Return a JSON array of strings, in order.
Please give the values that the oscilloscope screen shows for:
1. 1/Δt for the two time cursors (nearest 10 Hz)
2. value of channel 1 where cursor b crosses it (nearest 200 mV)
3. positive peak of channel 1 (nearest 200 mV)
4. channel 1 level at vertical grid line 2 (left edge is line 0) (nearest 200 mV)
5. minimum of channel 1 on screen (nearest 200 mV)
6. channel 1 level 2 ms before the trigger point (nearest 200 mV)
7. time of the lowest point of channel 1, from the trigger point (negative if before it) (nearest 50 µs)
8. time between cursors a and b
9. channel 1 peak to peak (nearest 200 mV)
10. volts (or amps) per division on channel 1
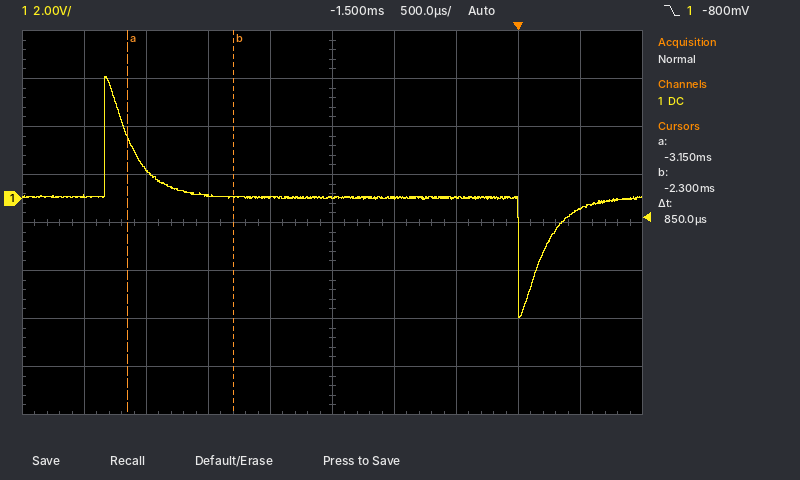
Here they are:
["1.18 kHz", "0.0 V", "5.0 V", "1.2 V", "-5.0 V", "0.0 V", "0 µs", "850 µs", "10.0 V", "2 V"]
